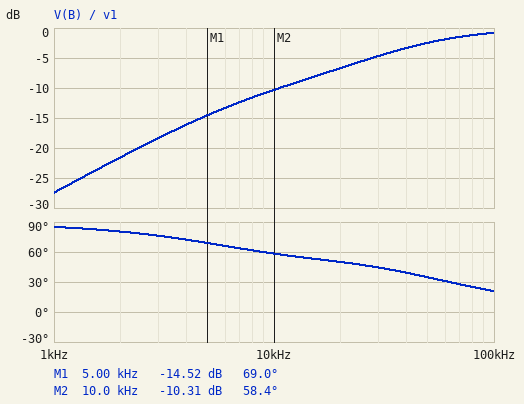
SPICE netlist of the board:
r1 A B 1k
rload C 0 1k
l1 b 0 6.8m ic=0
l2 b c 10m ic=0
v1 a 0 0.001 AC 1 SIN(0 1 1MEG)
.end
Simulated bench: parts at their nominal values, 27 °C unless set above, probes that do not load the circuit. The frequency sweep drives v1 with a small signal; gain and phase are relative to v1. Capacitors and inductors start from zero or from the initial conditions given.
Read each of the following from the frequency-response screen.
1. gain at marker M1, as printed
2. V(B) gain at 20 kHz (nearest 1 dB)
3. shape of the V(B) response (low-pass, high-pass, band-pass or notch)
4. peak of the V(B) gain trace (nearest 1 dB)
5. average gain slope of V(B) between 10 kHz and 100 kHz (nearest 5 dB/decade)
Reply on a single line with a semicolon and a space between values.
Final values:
-14.52 dB; -7 dB; high-pass; -1 dB; 10 dB/decade
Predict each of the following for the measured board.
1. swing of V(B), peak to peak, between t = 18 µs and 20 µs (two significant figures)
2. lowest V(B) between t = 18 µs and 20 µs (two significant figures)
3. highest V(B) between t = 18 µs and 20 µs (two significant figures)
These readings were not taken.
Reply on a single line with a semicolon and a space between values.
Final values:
2.0 V; -1.0 V; 1.0 V
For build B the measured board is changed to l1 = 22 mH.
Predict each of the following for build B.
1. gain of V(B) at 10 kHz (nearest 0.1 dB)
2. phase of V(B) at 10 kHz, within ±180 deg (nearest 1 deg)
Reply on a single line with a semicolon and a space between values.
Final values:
-6.4 dB; 34 deg
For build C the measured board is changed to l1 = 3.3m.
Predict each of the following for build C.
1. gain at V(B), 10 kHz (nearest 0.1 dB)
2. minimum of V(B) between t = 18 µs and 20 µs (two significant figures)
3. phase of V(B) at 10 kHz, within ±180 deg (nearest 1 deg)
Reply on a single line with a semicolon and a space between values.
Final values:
-14.9 dB; -1.0 V; 72 deg
